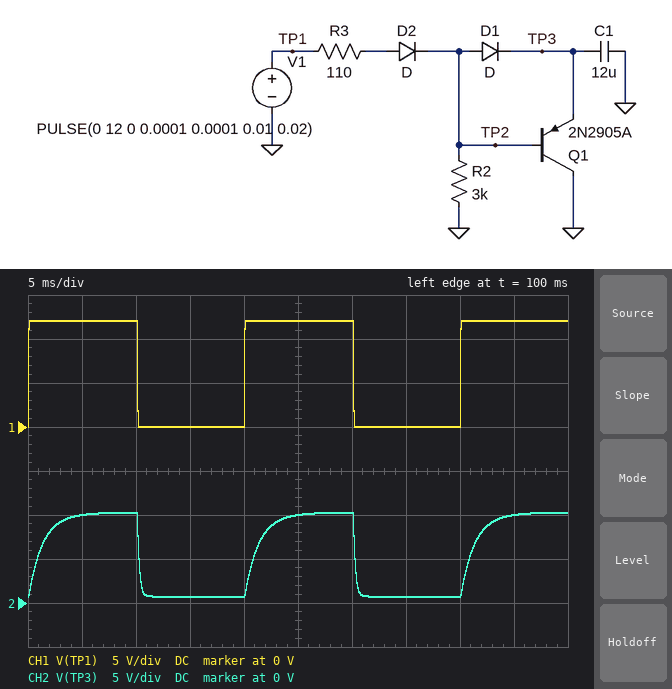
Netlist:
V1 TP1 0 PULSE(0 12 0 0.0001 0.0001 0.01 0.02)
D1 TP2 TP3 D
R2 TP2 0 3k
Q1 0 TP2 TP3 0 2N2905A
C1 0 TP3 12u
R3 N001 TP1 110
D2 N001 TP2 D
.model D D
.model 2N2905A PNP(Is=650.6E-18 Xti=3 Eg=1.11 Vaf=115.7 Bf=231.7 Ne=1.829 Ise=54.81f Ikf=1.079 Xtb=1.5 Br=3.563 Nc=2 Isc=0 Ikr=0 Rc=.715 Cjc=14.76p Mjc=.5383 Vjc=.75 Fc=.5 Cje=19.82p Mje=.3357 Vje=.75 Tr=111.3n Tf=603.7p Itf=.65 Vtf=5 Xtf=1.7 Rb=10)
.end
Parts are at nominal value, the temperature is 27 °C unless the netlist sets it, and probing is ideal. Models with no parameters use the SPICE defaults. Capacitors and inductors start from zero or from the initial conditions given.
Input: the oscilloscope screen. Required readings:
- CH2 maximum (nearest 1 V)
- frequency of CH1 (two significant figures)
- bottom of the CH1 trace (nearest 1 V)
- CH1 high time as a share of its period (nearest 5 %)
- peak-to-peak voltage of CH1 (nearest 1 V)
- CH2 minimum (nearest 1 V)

10 V
50 Hz
0 V
50 %
12 V
1 V
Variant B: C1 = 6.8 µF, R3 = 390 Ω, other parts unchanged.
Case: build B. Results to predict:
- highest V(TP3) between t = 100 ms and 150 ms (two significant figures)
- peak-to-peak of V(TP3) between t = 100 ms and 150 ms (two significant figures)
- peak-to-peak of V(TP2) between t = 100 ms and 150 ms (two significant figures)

9.2 V
8.6 V
9.9 V
